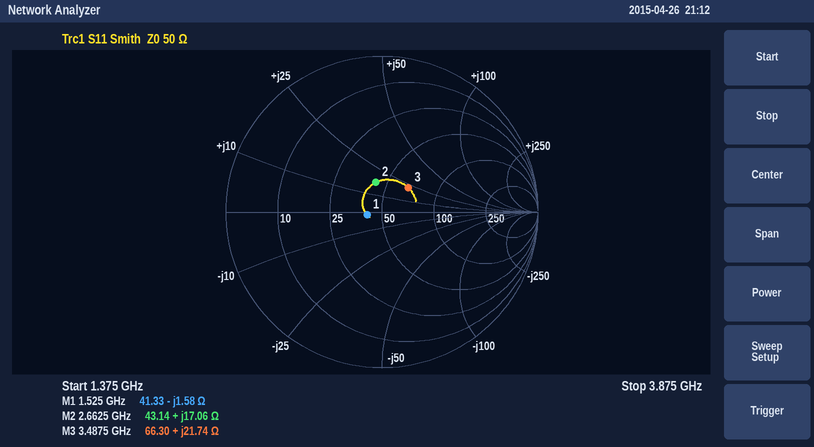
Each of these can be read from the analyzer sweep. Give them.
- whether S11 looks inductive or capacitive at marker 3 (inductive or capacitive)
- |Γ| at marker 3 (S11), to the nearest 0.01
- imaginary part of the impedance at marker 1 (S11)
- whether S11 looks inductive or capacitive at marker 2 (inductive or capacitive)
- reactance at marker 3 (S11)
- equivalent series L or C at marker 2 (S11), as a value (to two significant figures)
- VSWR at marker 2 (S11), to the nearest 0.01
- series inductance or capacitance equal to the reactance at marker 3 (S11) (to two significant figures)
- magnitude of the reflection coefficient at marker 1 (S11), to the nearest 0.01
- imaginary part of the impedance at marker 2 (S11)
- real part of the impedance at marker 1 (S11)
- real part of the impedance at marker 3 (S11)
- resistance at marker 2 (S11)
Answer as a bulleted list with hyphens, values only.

- inductive
- 0.23
- -1.58 Ω
- inductive
- +21.74 Ω
- 1.0 nH
- 1.48
- 990 pH
- 0.10
- +17.06 Ω
- 41.33 Ω
- 66.30 Ω
- 43.14 Ω
